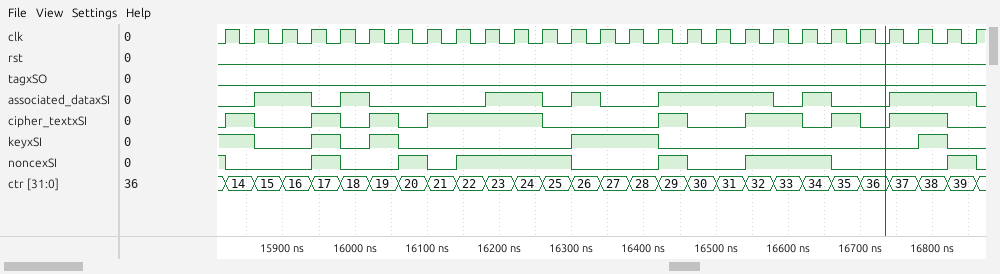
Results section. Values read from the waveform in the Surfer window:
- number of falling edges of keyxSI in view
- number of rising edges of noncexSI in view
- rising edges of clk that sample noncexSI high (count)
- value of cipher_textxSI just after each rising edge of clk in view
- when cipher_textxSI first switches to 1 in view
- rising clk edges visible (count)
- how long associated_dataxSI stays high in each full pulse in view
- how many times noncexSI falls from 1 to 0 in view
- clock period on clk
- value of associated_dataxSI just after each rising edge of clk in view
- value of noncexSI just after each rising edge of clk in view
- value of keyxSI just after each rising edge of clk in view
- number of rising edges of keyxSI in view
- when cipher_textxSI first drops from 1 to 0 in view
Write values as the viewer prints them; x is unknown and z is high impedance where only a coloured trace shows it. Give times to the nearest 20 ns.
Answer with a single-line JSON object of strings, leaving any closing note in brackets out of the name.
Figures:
{"number of falling edges of keyxSI in view": "5", "number of rising edges of noncexSI in view": "6", "rising edges of clk that sample noncexSI high": "12", "value of cipher_textxSI just after each rising edge of clk in view": "1 0 0 1 0 1 0 1 1 1 1 0 0 0 0 1 0 0 1 1 0 1 0 1 1 0 0", "when cipher_textxSI first switches to 1 in view": "15820 ns", "rising clk edges visible": "27", "how long associated_dataxSI stays high in each full pulse in view": "80 ns, 40 ns, 80 ns, 40 ns, 160 ns, 40 ns, 120 ns", "how many times noncexSI falls from 1 to 0 in view": "7", "clock period on clk": "40 ns", "value of associated_dataxSI just after each rising edge of clk in view": "0 1 1 0 1 0 0 0 0 1 1 0 1 0 0 1 1 1 1 0 1 0 0 1 1 1 0", "value of noncexSI just after each rising edge of clk in view": "0 0 0 1 0 0 1 0 1 1 1 1 0 0 0 1 0 0 1 1 1 0 0 0 0 1 0", "value of keyxSI just after each rising edge of clk in view": "1 0 0 1 0 1 0 0 0 0 0 0 1 1 1 0 0 0 0 0 0 0 0 0 1 0 0", "number of rising edges of keyxSI in view": "4", "when cipher_textxSI first drops from 1 to 0 in view": "15860 ns"}
